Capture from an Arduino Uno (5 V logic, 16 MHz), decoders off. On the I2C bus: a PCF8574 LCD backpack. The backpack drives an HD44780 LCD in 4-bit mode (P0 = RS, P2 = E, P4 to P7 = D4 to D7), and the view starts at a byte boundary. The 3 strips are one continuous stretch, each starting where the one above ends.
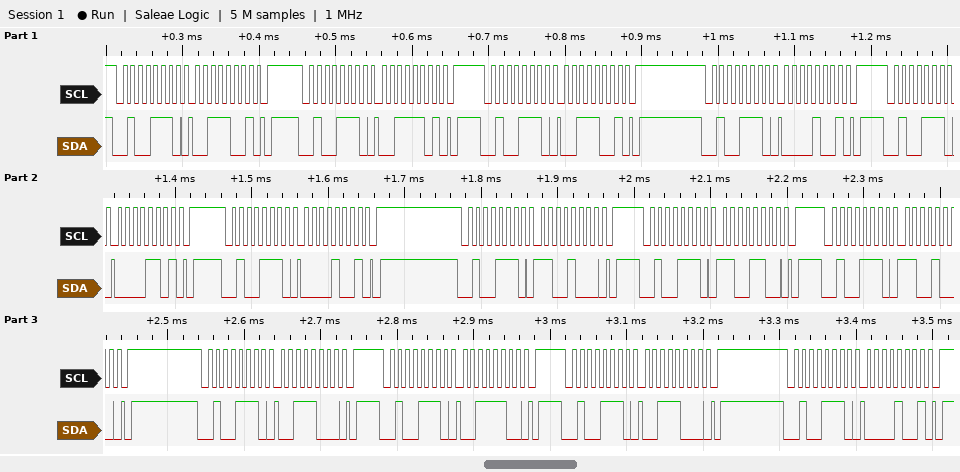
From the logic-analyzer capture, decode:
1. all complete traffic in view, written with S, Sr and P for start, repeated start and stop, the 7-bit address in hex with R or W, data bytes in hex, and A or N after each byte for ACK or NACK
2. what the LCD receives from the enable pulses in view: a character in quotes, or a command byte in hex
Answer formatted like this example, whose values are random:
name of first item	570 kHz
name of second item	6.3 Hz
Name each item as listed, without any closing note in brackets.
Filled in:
all complete traffic in view, written with S, Sr and P for start, repeated start and stop, the 7-bit address in hex with R or W, data bytes in hex, and A or N after each byte for ACK or NACK	S 27W A 39 A P S 27W A 3D A P S 27W A 39 A P S 27W A 09 A P S 27W A 0D A P S 27W A 09 A P S 27W A C8 A P S 27W A CC A P S 27W A C8 A P S 27W A 38 A P S 27W A 3C A P S 27W A 38 A P S 27W A 09 A P
what the LCD receives from the enable pulses in view: a character in quotes, or a command byte in hex	'0' 0xC3
